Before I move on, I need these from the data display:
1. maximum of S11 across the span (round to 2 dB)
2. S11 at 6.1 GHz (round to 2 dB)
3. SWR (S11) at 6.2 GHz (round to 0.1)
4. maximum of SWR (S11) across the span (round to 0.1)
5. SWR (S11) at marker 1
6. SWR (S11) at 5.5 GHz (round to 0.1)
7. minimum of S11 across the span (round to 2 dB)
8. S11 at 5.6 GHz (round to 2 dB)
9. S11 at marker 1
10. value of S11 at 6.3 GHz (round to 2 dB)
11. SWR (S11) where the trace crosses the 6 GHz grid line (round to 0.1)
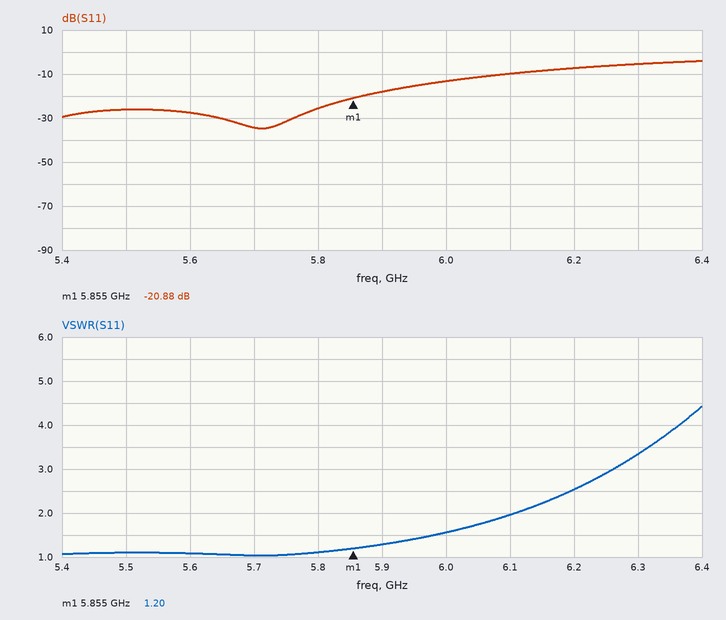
-4 dB
-10 dB
2.5
4.4
1.20
1.1
-34 dB
-28 dB
-20.88 dB
-6 dB
1.6
